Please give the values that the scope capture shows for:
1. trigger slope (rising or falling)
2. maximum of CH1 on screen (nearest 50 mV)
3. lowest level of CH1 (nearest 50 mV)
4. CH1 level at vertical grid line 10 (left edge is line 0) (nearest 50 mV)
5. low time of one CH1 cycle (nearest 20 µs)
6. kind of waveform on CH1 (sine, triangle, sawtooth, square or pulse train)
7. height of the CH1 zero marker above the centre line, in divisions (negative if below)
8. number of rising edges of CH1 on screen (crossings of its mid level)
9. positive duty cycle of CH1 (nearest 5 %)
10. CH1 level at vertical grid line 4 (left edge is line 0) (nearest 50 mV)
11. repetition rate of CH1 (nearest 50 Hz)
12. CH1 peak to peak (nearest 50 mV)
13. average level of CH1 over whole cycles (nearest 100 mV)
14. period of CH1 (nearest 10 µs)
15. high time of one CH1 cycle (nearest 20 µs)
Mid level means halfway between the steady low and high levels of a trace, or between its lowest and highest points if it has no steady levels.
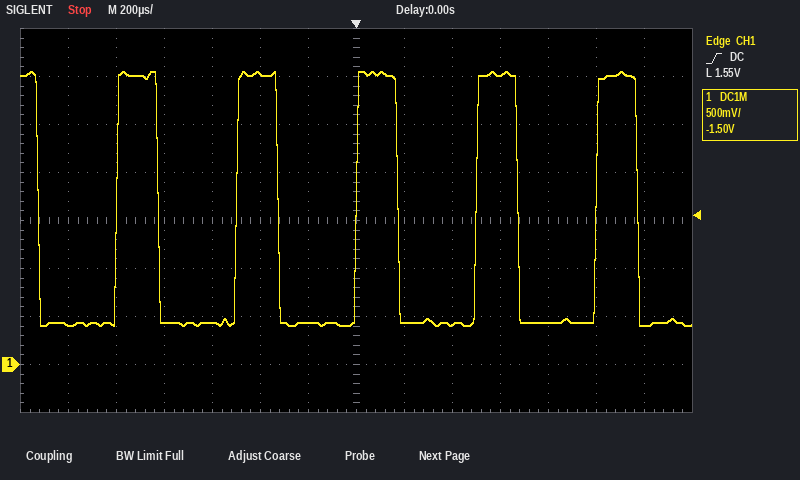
rising
3.05 V
400 mV
3.00 V
320 µs
pulse train
-3.0 div
5
35 %
450 mV
2.00 kHz
2.65 V
1.3 V
500 µs
180 µs
